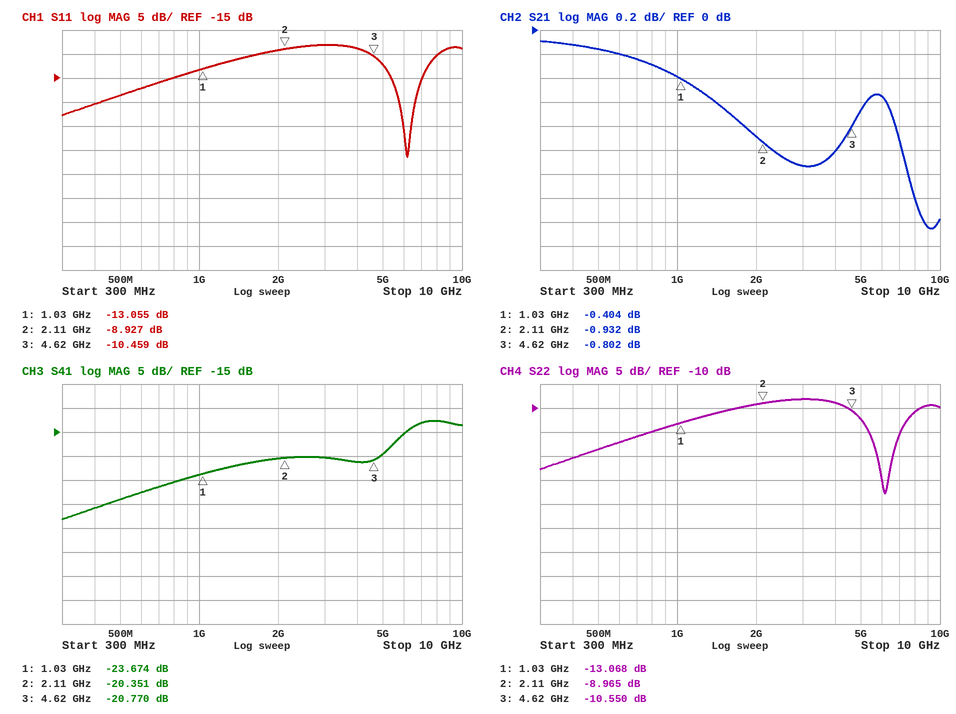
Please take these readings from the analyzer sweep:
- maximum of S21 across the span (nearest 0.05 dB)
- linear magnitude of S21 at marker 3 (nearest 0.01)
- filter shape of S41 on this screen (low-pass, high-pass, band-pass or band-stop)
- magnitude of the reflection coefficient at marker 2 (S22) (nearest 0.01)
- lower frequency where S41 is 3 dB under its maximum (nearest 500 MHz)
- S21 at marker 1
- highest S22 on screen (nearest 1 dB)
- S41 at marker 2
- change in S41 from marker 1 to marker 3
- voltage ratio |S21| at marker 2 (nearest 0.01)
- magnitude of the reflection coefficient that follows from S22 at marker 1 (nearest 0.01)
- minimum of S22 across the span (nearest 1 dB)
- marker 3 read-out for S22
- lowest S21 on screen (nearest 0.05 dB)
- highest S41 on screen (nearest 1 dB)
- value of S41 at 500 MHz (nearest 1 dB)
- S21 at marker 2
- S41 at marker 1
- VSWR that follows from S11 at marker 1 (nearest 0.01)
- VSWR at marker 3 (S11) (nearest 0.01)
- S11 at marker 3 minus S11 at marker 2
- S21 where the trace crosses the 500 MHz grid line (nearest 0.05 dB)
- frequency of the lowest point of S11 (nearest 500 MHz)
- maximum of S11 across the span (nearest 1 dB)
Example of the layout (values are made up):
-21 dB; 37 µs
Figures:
-0.10 dB; 0.91; high-pass; 0.36; 6.0 GHz; -0.404 dB; -8 dB; -20.351 dB; 2.904 dB; 0.90; 0.22; -28 dB; -10.550 dB; -1.65 dB; -13 dB; -29 dB; -0.932 dB; -23.674 dB; 1.57; 1.86; -1.532 dB; -0.15 dB; 6.0 GHz; -8 dB
